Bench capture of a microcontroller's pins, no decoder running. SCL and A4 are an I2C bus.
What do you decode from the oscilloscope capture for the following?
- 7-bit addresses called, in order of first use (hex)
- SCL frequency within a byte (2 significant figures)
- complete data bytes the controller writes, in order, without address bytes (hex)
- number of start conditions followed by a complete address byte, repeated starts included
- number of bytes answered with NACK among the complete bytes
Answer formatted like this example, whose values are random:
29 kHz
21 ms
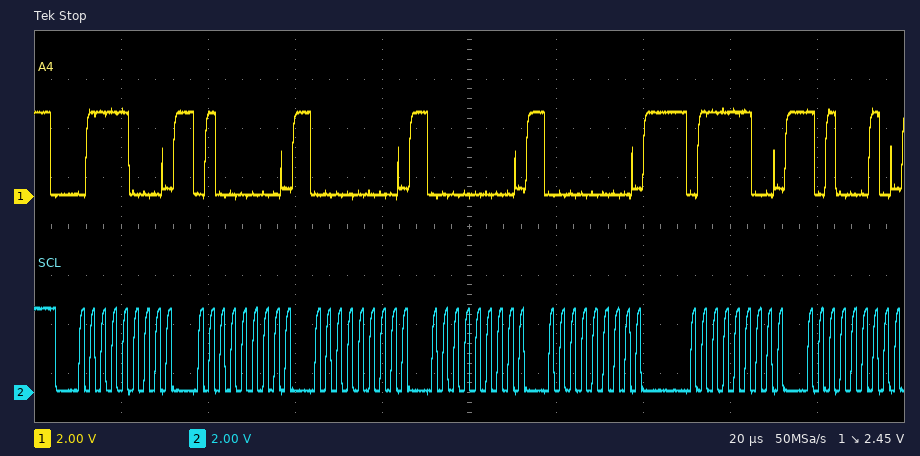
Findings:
0x3C
400 kHz
40 00 00 00 7C A2
1
0
